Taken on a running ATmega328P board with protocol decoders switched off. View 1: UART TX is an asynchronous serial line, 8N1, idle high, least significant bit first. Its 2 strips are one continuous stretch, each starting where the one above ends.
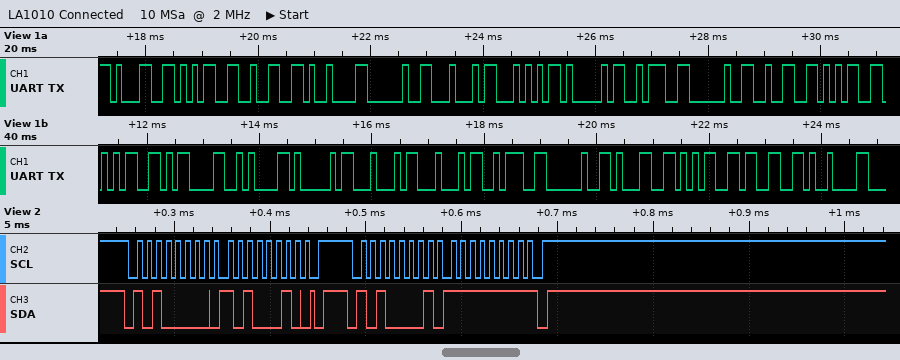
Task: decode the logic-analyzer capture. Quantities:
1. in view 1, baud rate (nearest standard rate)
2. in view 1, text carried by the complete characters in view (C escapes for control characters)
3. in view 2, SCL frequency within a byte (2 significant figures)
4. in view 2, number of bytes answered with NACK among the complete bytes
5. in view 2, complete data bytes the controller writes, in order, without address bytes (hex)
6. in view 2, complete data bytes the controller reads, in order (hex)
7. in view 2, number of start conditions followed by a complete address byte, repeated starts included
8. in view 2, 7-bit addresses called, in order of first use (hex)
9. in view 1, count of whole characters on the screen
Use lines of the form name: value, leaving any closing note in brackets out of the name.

in view 1, baud rate: 9600 baud
in view 1, text carried by the complete characters in view: "152\t DTA: 255\r\nADD: 153\t"
in view 2, SCL frequency within a byte: 100 kHz
in view 2, number of bytes answered with NACK among the complete bytes: 1
in view 2, complete data bytes the controller writes, in order, without address bytes: A2
in view 2, complete data bytes the controller reads, in order: FF
in view 2, number of start conditions followed by a complete address byte, repeated starts included: 2
in view 2, 7-bit addresses called, in order of first use: 0x50
in view 1, count of whole characters on the screen: 24
